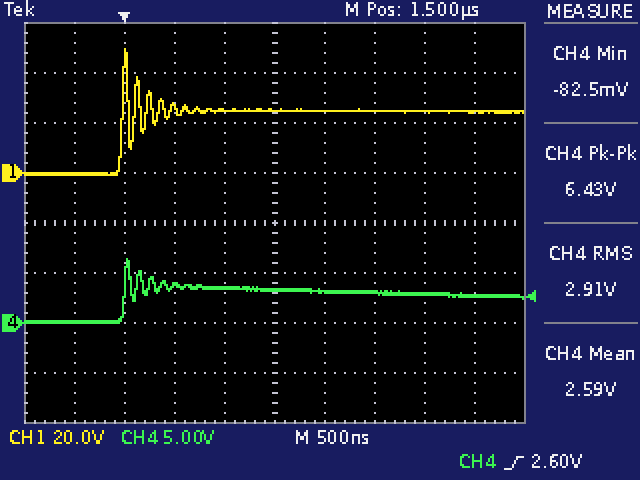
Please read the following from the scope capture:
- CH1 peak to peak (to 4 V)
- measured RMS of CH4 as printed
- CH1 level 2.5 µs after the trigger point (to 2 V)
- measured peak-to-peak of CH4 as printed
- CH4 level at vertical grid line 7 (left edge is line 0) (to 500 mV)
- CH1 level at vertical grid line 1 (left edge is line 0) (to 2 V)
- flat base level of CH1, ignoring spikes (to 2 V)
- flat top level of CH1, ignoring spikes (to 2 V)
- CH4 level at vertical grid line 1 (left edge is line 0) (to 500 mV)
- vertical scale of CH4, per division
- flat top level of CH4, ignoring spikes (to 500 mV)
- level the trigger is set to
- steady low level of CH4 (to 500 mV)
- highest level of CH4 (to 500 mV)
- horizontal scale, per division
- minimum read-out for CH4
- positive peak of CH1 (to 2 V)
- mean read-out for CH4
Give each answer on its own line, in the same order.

52 V
2.91 V
24 V
6.43 V
3.0 V
0 V
0 V
24 V
0.0 V
5 V
3.0 V
2.60 V
0.0 V
6.5 V
500 ns
-82.5 mV
50 V
2.59 V
